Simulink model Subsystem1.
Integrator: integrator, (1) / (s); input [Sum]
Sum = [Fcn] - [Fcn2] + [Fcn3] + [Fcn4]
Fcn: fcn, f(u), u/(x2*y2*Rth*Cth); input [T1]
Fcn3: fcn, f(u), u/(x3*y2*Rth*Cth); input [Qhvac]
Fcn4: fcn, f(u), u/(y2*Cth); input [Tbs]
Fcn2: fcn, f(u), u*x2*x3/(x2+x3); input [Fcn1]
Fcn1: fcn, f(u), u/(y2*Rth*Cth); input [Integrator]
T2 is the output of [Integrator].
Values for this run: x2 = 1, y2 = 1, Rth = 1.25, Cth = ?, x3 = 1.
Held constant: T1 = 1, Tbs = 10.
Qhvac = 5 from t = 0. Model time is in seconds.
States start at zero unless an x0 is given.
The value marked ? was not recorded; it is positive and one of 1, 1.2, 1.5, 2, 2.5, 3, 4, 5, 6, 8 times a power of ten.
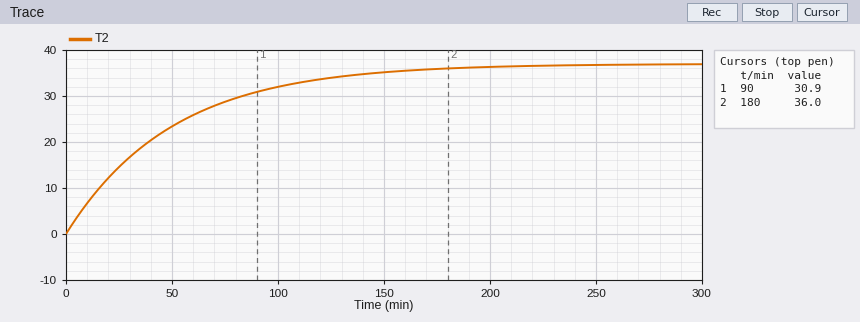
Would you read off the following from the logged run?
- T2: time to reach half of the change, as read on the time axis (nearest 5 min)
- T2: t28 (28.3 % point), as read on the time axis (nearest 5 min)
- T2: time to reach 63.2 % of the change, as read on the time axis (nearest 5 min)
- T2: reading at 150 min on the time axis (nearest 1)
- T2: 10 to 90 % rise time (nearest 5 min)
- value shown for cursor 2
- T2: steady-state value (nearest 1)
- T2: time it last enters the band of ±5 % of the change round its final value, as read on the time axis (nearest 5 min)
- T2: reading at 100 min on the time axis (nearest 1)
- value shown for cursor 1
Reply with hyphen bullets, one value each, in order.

- 35 min
- 15 min
- 50 min
- 35
- 110 min
- 36.0
- 37
- 150 min
- 32
- 30.9
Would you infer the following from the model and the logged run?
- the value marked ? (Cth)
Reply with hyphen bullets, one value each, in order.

- 1200
